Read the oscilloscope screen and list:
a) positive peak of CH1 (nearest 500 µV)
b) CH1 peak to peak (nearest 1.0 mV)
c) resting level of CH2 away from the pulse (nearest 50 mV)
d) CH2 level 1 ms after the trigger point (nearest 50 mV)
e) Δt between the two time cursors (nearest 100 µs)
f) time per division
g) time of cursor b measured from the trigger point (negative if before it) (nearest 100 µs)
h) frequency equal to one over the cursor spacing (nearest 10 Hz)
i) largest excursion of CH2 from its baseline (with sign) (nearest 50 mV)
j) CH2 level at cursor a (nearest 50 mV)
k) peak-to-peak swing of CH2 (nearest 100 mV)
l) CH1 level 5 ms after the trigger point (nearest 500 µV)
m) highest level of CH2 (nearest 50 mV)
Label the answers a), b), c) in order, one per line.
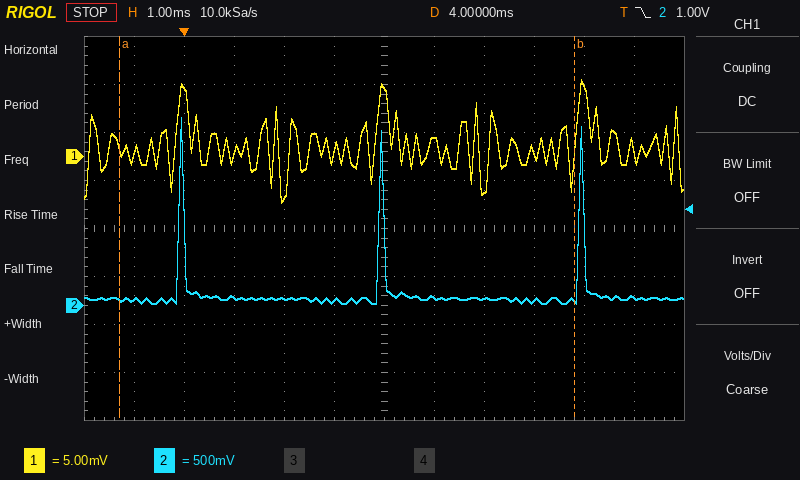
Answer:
a) 8.0 mV
b) 13.0 mV
c) 50 mV
d) 100 mV
e) 9.1 ms
f) 1 ms
g) +7.8 ms
h) 110 Hz
i) +1.90 V
j) 50 mV
k) 1.90 V
l) 2.0 mV
m) 1.95 V
